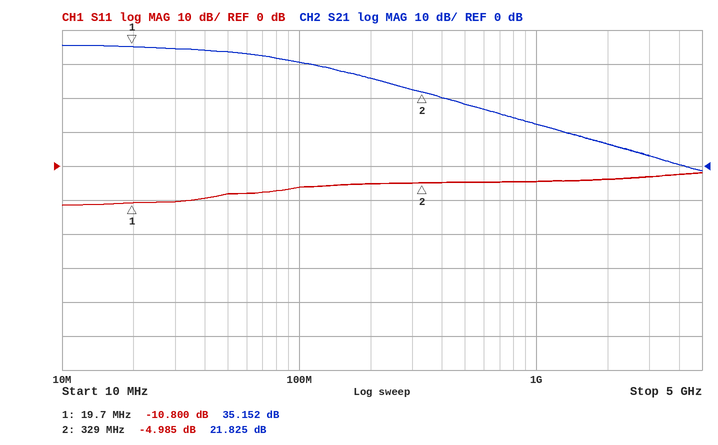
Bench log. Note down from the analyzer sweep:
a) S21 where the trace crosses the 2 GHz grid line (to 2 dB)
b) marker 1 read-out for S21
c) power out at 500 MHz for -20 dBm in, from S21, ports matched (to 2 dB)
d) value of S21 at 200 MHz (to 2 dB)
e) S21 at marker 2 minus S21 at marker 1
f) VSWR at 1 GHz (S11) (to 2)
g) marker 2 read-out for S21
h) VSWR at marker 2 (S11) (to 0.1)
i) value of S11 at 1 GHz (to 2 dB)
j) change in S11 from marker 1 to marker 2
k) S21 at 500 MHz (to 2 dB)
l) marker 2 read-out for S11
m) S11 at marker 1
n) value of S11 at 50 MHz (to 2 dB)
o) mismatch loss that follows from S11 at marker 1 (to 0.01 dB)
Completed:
6 dB
35.152 dB
-2 dBm
26 dB
-13.327 dB
4
21.825 dB
3.6
-4 dB
5.815 dB
18 dB
-4.985 dB
-10.800 dB
-8 dB
0.38 dB
